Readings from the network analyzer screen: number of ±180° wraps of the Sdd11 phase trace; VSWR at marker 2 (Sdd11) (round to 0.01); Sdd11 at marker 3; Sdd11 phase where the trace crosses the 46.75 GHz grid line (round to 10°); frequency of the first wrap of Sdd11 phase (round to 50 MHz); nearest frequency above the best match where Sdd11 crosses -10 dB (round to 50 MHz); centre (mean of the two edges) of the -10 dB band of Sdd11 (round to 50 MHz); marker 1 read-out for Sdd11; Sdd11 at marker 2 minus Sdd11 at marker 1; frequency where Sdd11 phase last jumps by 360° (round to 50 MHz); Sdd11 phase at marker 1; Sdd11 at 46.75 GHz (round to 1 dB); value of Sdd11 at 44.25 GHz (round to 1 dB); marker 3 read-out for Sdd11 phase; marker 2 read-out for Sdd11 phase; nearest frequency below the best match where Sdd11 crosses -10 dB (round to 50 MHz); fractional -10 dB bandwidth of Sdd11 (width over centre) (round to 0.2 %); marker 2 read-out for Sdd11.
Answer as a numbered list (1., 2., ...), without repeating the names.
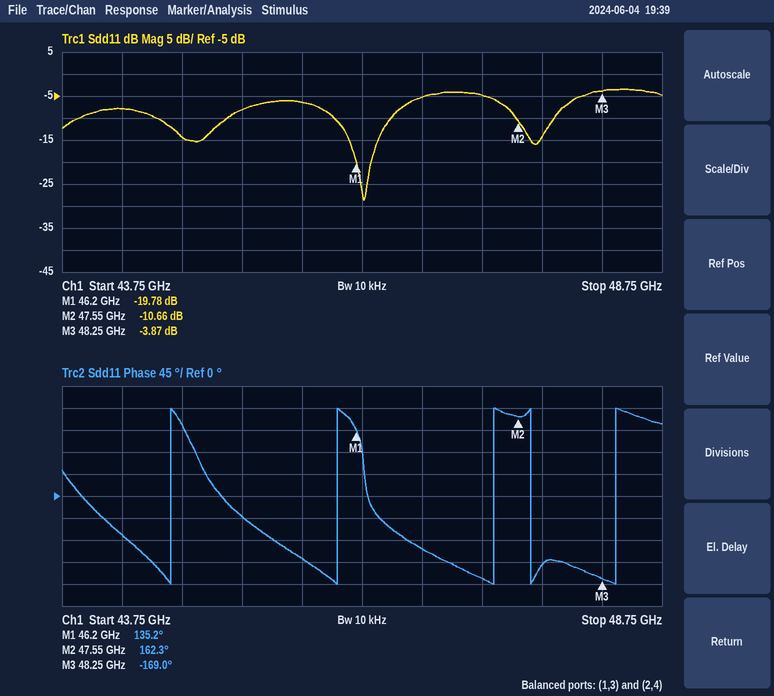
1. 5
2. 1.83
3. -3.87 dB
4. -110°
5. 44.65 GHz
6. 46.50 GHz
7. 46.25 GHz
8. -19.78 dB
9. 9.12 dB
10. 48.35 GHz
11. 135.2°
12. -5 dB
13. -8 dB
14. -169.0°
15. 162.3°
16. 46.00 GHz
17. 1.0 %
18. -10.66 dB
